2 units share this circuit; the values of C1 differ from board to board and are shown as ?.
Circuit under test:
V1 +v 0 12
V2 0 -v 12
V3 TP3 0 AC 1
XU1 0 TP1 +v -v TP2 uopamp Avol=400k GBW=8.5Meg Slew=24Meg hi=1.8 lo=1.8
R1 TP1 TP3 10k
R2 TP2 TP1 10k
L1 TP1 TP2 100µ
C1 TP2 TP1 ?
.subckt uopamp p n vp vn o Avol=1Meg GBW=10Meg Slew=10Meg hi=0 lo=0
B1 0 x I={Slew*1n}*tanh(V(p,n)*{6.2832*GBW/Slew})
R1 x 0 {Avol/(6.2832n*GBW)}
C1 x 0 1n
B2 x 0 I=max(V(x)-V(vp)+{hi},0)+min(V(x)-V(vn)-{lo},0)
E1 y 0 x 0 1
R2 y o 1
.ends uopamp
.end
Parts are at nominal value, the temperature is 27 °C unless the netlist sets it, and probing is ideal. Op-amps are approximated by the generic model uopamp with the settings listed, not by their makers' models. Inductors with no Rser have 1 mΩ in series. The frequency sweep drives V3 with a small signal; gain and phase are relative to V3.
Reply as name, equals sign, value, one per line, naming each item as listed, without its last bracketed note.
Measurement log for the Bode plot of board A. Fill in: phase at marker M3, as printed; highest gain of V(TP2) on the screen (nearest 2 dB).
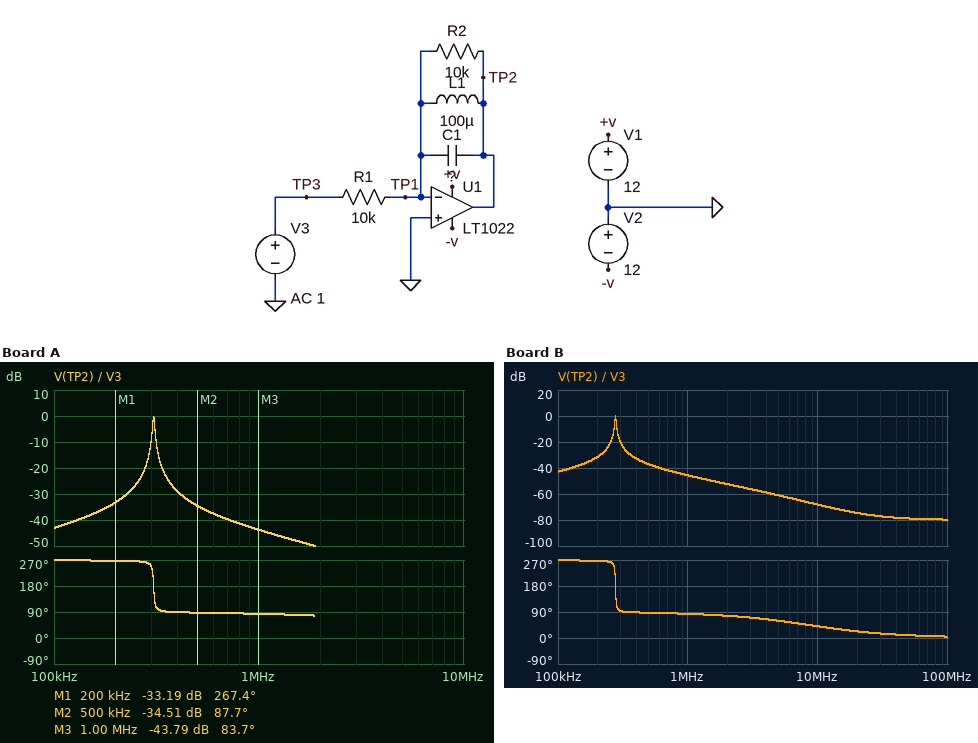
phase at marker M3, as printed = 83.7 deg
highest gain of V(TP2) on the screen = 0 dB
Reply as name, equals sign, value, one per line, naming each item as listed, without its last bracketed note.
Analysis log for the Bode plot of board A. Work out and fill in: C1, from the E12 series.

C1, from the E12 series = 2.7 nF
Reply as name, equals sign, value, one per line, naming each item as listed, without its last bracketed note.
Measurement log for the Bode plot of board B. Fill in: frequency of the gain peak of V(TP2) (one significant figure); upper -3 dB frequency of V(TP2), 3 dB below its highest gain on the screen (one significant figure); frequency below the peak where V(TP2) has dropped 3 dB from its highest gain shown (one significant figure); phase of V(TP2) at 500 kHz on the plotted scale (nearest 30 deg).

frequency of the gain peak of V(TP2) = 300 kHz
upper -3 dB frequency of V(TP2), 3 dB below its highest gain on the screen = 300 kHz
frequency below the peak where V(TP2) has dropped 3 dB from its highest gain shown = 300 kHz
phase of V(TP2) at 500 kHz on the plotted scale = 90 deg
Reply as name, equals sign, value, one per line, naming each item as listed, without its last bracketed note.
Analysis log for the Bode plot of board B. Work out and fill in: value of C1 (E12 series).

value of C1 = 3.3 nF
